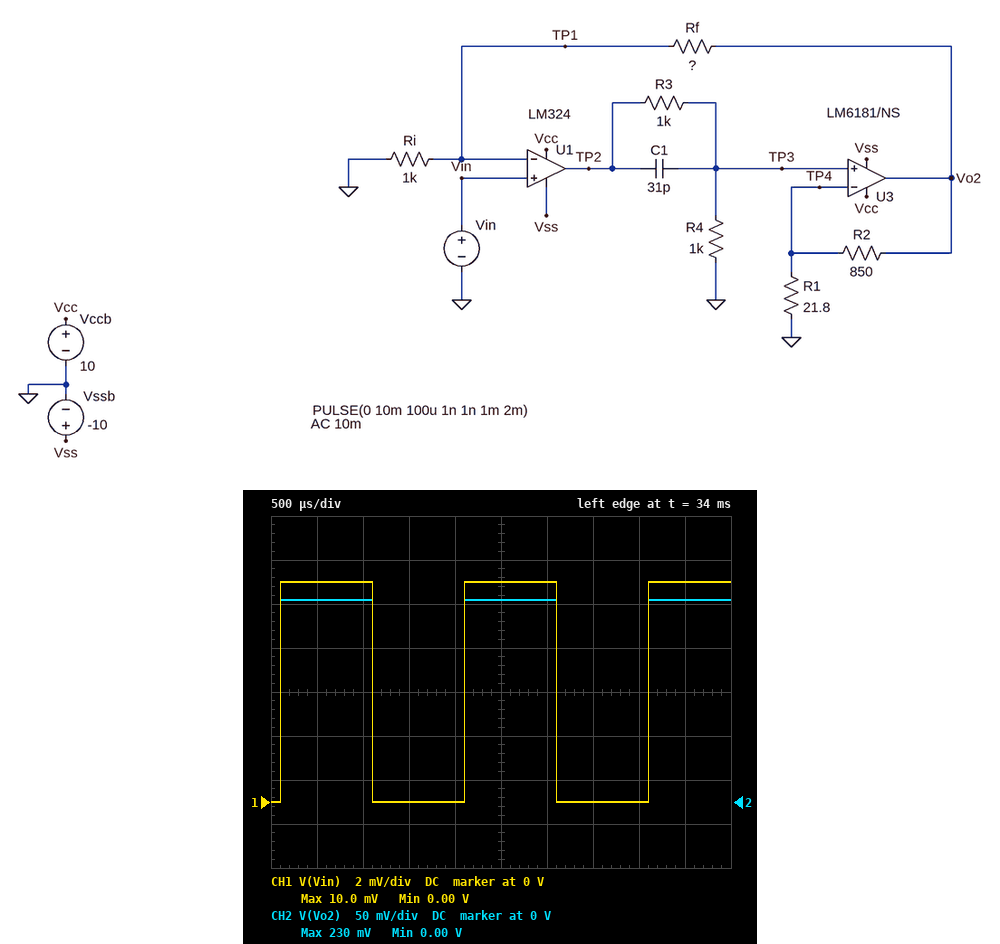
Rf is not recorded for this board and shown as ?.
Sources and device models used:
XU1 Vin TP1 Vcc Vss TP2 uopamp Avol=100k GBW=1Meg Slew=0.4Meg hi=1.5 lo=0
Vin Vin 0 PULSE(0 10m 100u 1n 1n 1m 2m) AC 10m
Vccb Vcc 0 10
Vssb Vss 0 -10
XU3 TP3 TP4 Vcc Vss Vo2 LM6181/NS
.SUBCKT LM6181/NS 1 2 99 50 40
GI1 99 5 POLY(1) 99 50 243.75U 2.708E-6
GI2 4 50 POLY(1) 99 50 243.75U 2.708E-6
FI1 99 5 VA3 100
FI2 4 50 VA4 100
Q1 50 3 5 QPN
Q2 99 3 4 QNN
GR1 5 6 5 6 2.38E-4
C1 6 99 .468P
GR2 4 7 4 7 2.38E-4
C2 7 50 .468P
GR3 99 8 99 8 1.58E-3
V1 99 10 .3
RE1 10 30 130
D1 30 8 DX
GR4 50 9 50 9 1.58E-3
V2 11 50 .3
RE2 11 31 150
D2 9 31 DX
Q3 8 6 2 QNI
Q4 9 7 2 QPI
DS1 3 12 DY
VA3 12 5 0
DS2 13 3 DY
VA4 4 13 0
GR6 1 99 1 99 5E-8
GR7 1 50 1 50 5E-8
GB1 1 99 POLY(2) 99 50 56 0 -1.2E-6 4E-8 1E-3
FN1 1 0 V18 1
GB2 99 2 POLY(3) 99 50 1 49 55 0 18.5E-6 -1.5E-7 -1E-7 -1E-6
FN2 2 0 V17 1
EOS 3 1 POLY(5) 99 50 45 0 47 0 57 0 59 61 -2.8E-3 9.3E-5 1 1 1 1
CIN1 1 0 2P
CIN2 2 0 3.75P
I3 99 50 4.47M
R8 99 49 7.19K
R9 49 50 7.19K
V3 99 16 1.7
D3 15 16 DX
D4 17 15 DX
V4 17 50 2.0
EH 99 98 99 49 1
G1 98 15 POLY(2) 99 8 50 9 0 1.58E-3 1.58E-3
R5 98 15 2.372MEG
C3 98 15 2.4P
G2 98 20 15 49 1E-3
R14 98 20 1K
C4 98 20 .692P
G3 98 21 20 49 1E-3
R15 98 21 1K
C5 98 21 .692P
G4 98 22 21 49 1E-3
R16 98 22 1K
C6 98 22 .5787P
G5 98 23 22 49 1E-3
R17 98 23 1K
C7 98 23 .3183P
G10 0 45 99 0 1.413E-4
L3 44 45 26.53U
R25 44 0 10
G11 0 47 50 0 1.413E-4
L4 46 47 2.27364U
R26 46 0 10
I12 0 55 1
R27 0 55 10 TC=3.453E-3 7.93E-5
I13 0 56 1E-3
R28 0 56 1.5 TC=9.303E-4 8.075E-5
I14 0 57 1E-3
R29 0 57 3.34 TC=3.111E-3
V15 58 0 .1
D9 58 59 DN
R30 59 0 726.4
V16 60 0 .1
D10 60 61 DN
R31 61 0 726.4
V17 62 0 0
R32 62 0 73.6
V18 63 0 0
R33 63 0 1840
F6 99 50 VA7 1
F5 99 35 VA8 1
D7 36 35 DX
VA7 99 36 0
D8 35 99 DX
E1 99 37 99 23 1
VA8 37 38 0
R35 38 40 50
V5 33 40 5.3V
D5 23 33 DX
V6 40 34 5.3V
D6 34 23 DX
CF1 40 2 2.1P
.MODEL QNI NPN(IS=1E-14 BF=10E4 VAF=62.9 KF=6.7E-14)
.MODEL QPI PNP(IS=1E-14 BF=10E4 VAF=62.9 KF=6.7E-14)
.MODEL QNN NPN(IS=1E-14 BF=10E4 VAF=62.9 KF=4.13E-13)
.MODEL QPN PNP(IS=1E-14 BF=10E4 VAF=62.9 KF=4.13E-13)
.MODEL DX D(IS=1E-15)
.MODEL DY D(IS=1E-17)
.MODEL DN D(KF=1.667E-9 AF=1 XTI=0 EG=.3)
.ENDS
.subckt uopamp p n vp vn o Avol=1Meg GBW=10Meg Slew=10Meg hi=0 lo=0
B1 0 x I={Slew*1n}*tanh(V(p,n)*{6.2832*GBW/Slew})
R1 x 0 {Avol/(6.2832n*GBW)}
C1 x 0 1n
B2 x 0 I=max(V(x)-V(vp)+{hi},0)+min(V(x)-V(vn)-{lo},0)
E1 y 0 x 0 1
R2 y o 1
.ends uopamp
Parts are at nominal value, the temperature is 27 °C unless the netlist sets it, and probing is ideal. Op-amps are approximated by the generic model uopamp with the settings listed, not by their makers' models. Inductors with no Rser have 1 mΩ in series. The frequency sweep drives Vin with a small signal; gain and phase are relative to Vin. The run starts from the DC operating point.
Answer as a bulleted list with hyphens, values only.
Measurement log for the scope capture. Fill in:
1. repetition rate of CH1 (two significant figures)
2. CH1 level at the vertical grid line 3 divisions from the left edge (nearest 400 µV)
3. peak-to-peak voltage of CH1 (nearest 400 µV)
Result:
- 500 Hz
- 0 V
- 10.0 mV
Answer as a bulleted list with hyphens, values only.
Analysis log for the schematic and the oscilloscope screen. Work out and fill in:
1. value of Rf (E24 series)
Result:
- 22 kΩ
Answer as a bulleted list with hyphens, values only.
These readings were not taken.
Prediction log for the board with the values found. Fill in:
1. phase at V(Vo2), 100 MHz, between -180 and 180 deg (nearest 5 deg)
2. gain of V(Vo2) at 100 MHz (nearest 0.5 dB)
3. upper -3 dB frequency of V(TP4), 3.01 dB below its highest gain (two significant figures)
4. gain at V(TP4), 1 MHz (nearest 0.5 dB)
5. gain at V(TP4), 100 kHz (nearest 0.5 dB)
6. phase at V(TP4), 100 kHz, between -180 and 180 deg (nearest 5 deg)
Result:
- 65 deg
- -26.0 dB
- 860 kHz
- -8.5 dB
- -5.0 dB
- -5 deg
